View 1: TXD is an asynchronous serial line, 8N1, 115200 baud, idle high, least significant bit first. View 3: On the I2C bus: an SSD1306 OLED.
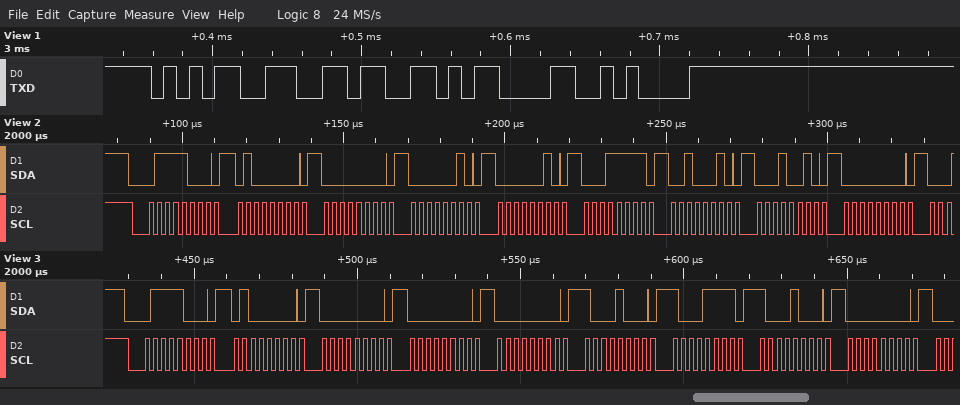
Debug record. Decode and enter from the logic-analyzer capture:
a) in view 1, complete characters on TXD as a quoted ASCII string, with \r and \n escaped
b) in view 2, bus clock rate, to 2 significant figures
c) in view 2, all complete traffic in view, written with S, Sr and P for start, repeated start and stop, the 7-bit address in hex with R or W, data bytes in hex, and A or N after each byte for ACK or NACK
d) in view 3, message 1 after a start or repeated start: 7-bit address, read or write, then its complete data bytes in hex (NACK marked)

"56\r\n"
400 kHz
S 3CW A 40 A 00 A 02 A 02 A 1F A 22 A 12 A 00 A
0x3C write: 40 00 00 00 88 8F 88 00
